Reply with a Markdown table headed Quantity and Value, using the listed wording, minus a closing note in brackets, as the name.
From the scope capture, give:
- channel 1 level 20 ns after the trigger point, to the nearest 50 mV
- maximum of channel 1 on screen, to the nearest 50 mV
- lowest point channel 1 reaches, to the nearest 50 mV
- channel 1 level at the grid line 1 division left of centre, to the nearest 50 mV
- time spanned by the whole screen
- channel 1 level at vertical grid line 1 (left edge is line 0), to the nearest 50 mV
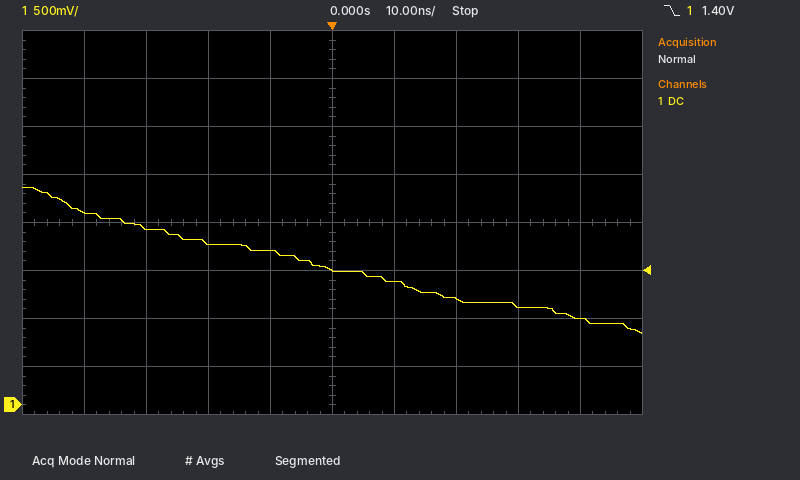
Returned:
| Quantity | Value |
|---|---|
| channel 1 level 20 ns after the trigger point, to the nearest 50 mV | 1.10 V |
| maximum of channel 1 on screen, to the nearest 50 mV | 2.25 V |
| lowest point channel 1 reaches, to the nearest 50 mV | 750 mV |
| channel 1 level at the grid line 1 division left of centre, to the nearest 50 mV | 1.60 V |
| time spanned by the whole screen | 100 ns |
| channel 1 level at vertical grid line 1 (left edge is line 0), to the nearest 50 mV | 2.00 V |
